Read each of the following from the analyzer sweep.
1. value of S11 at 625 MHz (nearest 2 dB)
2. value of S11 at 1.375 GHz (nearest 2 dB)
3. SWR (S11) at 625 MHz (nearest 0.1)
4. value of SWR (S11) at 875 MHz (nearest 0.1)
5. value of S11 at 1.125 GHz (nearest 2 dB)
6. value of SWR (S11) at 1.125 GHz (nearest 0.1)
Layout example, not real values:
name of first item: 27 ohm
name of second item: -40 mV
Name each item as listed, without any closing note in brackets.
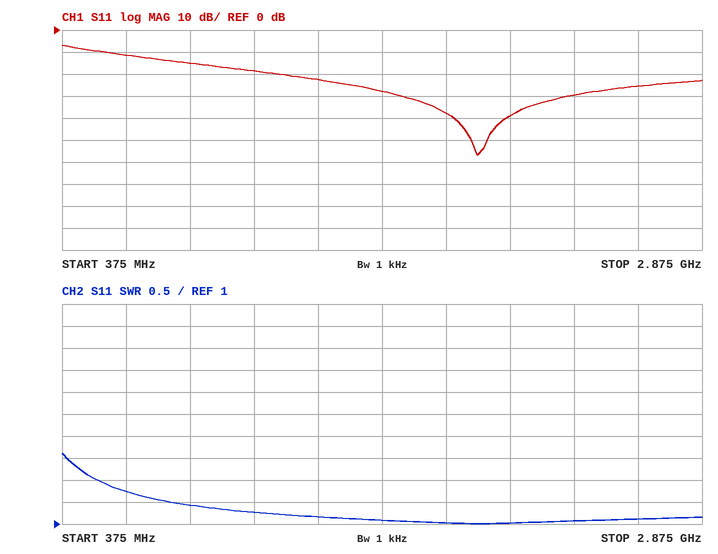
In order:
value of S11 at 625 MHz: -12 dB
value of S11 at 1.375 GHz: -22 dB
SWR (S11) at 625 MHz: 1.7
value of SWR (S11) at 875 MHz: 1.4
value of S11 at 1.125 GHz: -18 dB
value of SWR (S11) at 1.125 GHz: 1.3
